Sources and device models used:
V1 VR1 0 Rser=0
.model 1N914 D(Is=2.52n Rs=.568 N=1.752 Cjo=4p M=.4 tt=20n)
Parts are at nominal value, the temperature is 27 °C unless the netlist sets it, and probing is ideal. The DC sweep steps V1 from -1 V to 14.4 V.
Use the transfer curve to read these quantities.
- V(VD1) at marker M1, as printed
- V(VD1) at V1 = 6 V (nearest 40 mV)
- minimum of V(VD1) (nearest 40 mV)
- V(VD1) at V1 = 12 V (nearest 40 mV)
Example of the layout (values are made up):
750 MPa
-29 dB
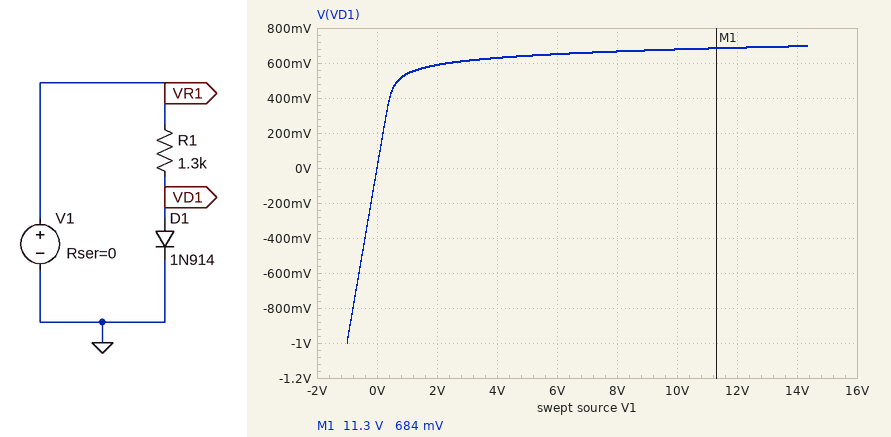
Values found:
684 mV
640 mV
-1.00 V
680 mV
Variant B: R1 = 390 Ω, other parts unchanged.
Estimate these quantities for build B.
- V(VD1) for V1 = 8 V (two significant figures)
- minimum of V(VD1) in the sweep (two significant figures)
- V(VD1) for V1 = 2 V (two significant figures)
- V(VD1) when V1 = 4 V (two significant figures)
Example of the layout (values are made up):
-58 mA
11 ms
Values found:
730 mV
-1.0 V
640 mV
690 mV
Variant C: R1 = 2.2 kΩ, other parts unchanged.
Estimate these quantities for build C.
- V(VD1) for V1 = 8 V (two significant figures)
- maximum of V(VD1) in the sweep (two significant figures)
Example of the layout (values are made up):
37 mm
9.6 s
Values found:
640 mV
670 mV
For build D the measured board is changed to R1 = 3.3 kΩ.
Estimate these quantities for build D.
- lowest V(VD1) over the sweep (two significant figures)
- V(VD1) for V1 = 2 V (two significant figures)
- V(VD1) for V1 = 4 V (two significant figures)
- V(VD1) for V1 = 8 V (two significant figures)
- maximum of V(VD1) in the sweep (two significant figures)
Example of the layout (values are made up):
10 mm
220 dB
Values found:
-1.0 V
550 mV
590 mV
620 mV
650 mV
